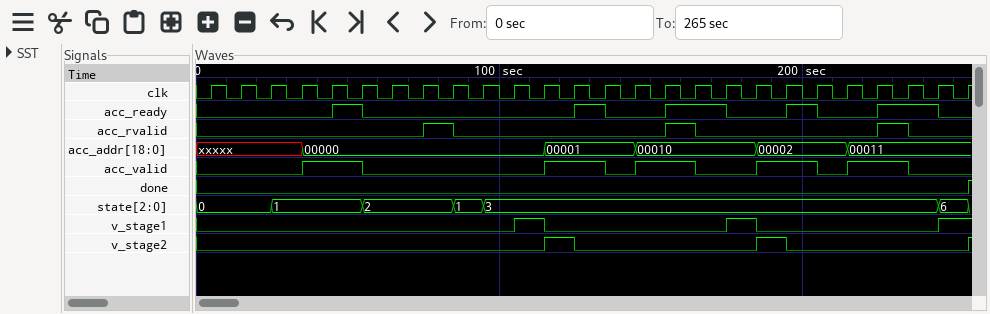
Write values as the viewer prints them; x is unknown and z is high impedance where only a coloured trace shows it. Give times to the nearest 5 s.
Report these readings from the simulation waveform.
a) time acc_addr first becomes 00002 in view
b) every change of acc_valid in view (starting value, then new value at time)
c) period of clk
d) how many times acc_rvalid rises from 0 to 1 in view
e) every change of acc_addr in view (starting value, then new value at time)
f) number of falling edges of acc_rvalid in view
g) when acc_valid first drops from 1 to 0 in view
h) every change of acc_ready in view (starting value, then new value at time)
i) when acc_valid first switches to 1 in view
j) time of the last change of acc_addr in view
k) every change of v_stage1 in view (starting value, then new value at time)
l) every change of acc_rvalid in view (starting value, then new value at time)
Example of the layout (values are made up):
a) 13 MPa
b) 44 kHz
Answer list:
a) 185 s
b) 0, 1 at 35 s, 0 at 55 s, 1 at 115 s, 0 at 135 s, 1 at 145 s, 0 at 165 s, 1 at 185 s, 0 at 205 s, 1 at 215 s, 0 at 235 s
c) 10 s
d) 3
e) xxxxx, 00000 at 35 s, 00001 at 115 s, 00010 at 145 s, 00002 at 185 s, 00011 at 215 s
f) 3
g) 55 s
h) 0, 1 at 45 s, 0 at 55 s, 1 at 125 s, 0 at 135 s, 1 at 155 s, 0 at 175 s, 1 at 195 s, 0 at 205 s, 1 at 225 s, 0 at 245 s
i) 35 s
j) 215 s
k) 0, 1 at 105 s, 0 at 115 s, 1 at 175 s, 0 at 185 s, 1 at 245 s
l) 0, 1 at 75 s, 0 at 85 s, 1 at 155 s, 0 at 165 s, 1 at 225 s, 0 at 235 s
